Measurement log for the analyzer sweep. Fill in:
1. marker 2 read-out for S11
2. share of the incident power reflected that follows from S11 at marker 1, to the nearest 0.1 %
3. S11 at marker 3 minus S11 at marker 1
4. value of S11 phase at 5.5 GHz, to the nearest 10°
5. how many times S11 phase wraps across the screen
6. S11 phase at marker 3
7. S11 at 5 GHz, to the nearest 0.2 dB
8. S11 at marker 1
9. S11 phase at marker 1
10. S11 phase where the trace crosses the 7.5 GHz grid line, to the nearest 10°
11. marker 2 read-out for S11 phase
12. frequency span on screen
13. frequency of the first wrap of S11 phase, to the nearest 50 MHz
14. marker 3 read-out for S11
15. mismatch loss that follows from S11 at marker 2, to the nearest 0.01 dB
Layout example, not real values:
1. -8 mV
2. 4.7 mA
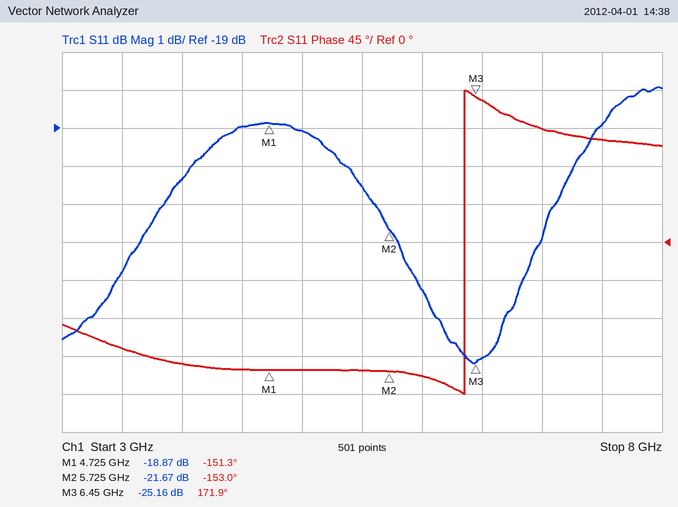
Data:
1. -21.67 dB
2. 1.3 %
3. -6.29 dB
4. -150°
5. 1
6. 171.9°
7. -19.0 dB
8. -18.87 dB
9. -151.3°
10. 120°
11. -153.0°
12. 5 GHz
13. 6.35 GHz
14. -25.16 dB
15. 0.03 dB
